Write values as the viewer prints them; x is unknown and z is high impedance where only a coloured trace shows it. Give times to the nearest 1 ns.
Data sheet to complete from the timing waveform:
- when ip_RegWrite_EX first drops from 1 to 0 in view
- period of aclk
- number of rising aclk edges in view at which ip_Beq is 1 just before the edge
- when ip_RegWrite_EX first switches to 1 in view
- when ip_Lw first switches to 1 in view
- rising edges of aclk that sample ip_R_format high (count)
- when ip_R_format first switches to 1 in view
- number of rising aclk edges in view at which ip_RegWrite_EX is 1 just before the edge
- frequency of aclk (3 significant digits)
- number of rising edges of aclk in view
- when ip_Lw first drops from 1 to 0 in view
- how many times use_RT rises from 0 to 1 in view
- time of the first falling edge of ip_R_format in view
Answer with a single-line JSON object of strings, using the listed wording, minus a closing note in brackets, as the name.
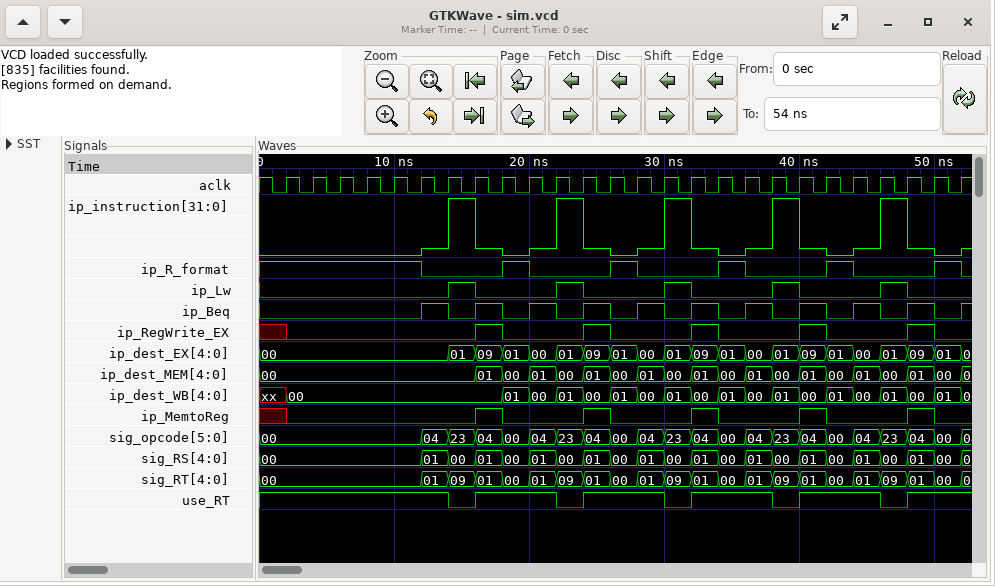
{"when ip_RegWrite_EX first drops from 1 to 0 in view": "18 ns", "period of aclk": "2 ns", "number of rising aclk edges in view at which ip_Beq is 1 just before the edge": "10", "when ip_RegWrite_EX first switches to 1 in view": "16 ns", "when ip_Lw first switches to 1 in view": "14 ns", "rising edges of aclk that sample ip_R_format high": "11", "when ip_R_format first switches to 1 in view": "18 ns", "number of rising aclk edges in view at which ip_RegWrite_EX is 1 just before the edge": "5", "frequency of aclk": "500 MHz", "number of rising edges of aclk in view": "26", "when ip_Lw first drops from 1 to 0 in view": "16 ns", "how many times use_RT rises from 0 to 1 in view": "5", "time of the first falling edge of ip_R_format in view": "12 ns"}
